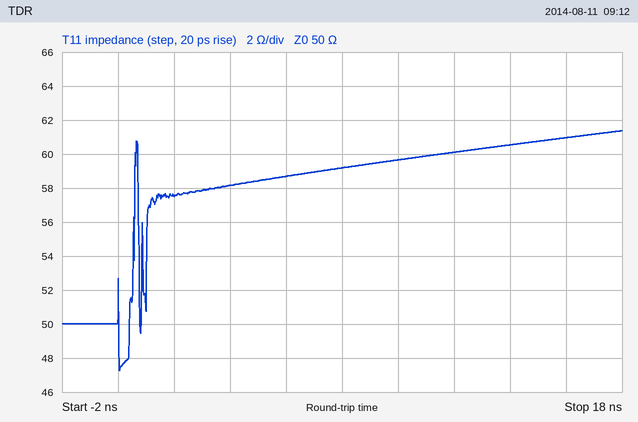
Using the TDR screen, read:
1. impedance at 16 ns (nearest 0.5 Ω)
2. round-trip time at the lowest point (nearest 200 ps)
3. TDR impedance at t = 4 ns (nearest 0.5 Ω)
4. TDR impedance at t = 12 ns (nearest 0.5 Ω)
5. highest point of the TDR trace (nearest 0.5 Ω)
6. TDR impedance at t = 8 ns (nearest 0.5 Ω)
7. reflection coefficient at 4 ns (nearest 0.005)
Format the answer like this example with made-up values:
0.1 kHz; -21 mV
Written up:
61.0 Ω; 0.0 ns; 58.0 Ω; 60.0 Ω; 61.5 Ω; 59.0 Ω; +0.075
